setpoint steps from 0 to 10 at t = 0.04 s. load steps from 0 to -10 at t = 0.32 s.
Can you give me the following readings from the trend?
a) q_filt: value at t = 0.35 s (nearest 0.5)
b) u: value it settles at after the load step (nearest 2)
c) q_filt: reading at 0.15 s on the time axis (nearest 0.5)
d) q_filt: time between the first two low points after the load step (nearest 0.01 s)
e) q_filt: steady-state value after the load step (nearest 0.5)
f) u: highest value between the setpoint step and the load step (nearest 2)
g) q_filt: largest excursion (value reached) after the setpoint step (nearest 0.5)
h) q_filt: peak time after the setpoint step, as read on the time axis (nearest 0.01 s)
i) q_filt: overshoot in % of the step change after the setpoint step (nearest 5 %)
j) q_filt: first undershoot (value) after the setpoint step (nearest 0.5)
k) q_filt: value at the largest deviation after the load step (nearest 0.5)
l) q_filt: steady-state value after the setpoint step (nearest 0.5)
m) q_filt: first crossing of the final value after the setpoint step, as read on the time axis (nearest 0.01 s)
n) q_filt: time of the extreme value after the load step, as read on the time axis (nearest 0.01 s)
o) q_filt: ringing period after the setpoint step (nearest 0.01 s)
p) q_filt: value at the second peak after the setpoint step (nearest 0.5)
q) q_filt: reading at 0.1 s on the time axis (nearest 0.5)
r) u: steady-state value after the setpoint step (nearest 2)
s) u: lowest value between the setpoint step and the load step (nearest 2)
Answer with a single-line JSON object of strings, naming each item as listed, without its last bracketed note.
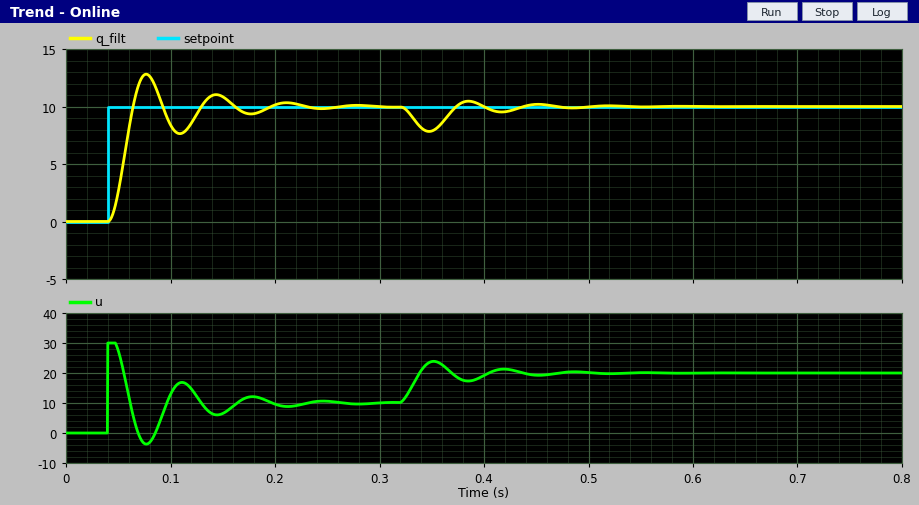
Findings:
{"q_filt: value at t = 0.35 s": "8.0", "u: value it settles at after the load step": "20", "q_filt: reading at 0.15 s on the time axis": "11.0", "q_filt: time between the first two low points after the load step": "0.07 s", "q_filt: steady-state value after the load step": "10.0", "u: highest value between the setpoint step and the load step": "30", "q_filt: largest excursion (value reached) after the setpoint step": "13.0", "q_filt: peak time after the setpoint step, as read on the time axis": "0.08 s", "q_filt: overshoot in % of the step change after the setpoint step": "30 %", "q_filt: first undershoot (value) after the setpoint step": "7.5", "q_filt: value at the largest deviation after the load step": "8.0", "q_filt: steady-state value after the setpoint step": "10.0", "q_filt: first crossing of the final value after the setpoint step, as read on the time axis": "0.06 s", "q_filt: time of the extreme value after the load step, as read on the time axis": "0.35 s", "q_filt: ringing period after the setpoint step": "0.07 s", "q_filt: value at the second peak after the setpoint step": "11.0", "q_filt: reading at 0.1 s on the time axis": "8.5", "u: steady-state value after the setpoint step": "10", "u: lowest value between the setpoint step and the load step": "-4"}
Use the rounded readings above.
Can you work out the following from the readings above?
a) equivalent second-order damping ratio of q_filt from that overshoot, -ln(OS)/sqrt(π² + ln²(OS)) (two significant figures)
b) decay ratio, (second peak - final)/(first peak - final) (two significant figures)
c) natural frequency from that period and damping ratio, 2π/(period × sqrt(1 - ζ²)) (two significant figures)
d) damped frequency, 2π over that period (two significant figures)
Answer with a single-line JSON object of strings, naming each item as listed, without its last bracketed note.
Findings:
{"equivalent second-order damping ratio of q_filt from that overshoot, -ln(OS)/sqrt(π² + ln²(OS))": "0.36", "decay ratio, (second peak - final)/(first peak - final)": "0.33", "natural frequency from that period and damping ratio, 2π/(period × sqrt(1 - ζ²))": "96 rad/s", "damped frequency, 2π over that period": "90 rad/s"}
